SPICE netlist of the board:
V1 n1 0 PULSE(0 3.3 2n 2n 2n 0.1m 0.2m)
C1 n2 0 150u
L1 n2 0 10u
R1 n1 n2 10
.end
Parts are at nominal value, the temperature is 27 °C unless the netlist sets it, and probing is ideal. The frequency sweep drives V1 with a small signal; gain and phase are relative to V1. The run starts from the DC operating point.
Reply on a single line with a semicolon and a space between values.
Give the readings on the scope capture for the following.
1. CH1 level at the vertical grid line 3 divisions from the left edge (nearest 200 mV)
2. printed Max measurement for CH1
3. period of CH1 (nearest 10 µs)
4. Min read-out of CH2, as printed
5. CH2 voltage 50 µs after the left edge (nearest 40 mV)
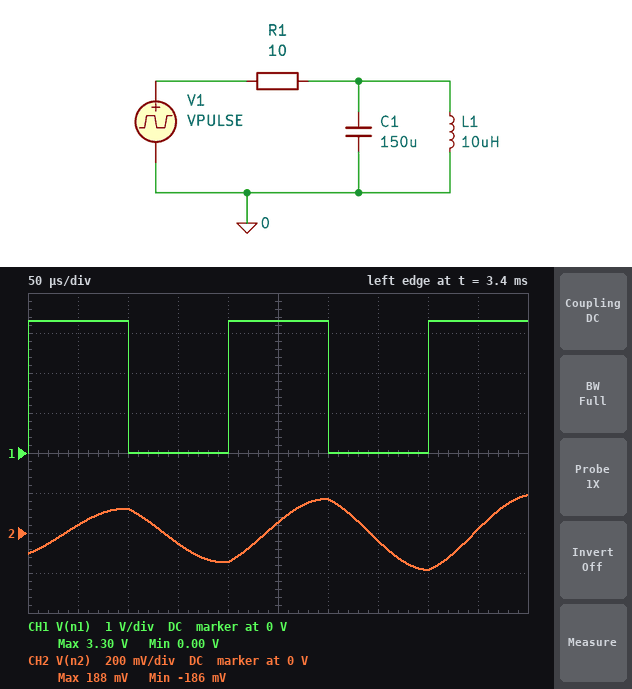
0 V; 3.30 V; 200 µs; -186 mV; 40 mV
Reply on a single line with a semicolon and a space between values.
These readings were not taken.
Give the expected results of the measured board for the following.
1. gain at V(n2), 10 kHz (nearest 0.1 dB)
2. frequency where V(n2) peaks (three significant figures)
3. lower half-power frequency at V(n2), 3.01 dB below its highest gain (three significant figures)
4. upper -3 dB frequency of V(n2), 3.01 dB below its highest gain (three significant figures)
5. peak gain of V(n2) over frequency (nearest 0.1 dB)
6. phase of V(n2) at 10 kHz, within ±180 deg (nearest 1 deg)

-37.9 dB; 4.11 kHz; 4.06 kHz; 4.16 kHz; 0 dB; -89 deg
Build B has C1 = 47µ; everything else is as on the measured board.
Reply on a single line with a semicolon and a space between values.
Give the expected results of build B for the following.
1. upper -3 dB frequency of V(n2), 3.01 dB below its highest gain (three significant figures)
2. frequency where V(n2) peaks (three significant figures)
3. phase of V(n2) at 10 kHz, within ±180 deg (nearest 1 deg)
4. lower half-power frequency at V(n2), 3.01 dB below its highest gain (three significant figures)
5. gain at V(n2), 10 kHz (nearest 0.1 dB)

7.51 kHz; 7.34 kHz; -86 deg; 7.17 kHz; -22.7 dB
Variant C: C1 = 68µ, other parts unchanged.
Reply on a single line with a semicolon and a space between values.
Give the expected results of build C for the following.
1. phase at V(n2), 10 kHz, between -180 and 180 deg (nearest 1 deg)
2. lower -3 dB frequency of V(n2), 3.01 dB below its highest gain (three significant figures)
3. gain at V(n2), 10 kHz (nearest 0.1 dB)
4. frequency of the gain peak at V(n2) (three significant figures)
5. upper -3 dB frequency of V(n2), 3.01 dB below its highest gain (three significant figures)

-88 deg; 5.99 kHz; -28.6 dB; 6.10 kHz; 6.22 kHz
